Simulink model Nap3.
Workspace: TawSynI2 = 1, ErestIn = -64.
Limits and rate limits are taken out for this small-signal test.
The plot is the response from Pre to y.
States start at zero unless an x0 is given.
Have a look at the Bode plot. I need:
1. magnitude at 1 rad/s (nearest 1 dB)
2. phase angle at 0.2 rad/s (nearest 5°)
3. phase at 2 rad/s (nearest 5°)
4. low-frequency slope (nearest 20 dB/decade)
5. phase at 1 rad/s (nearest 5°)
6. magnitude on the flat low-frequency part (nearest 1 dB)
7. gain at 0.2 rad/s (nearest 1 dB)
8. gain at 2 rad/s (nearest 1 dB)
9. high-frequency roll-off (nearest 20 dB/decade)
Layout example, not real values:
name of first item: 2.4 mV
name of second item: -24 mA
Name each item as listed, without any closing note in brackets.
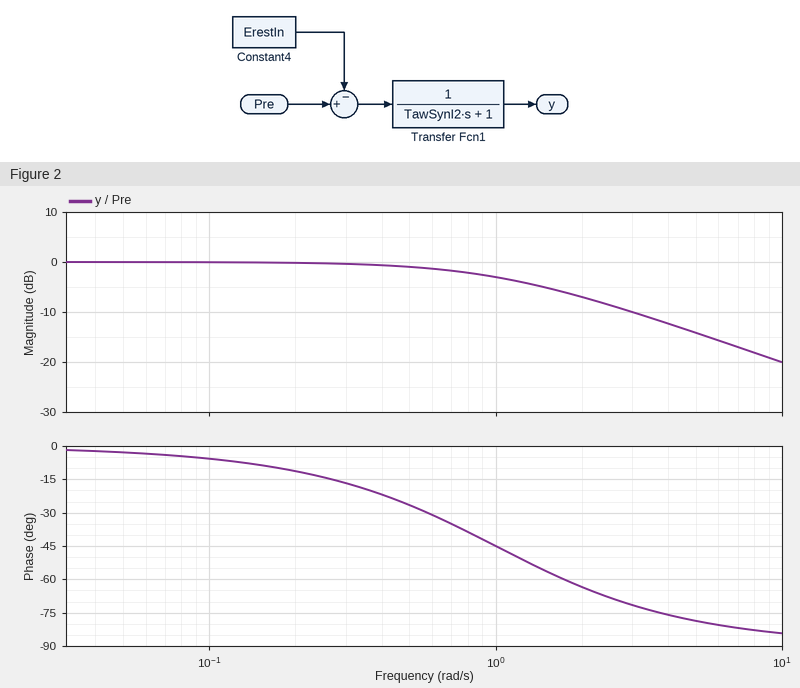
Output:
magnitude at 1 rad/s: -3 dB
phase angle at 0.2 rad/s: -10°
phase at 2 rad/s: -65°
low-frequency slope: 0 dB/decade
phase at 1 rad/s: -45°
magnitude on the flat low-frequency part: 0 dB
gain at 0.2 rad/s: 0 dB
gain at 2 rad/s: -7 dB
high-frequency roll-off: -20 dB/decade
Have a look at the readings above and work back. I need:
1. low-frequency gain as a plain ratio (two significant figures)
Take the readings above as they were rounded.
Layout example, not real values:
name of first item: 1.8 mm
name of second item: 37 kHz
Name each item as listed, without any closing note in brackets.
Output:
low-frequency gain as a plain ratio: 1.0
